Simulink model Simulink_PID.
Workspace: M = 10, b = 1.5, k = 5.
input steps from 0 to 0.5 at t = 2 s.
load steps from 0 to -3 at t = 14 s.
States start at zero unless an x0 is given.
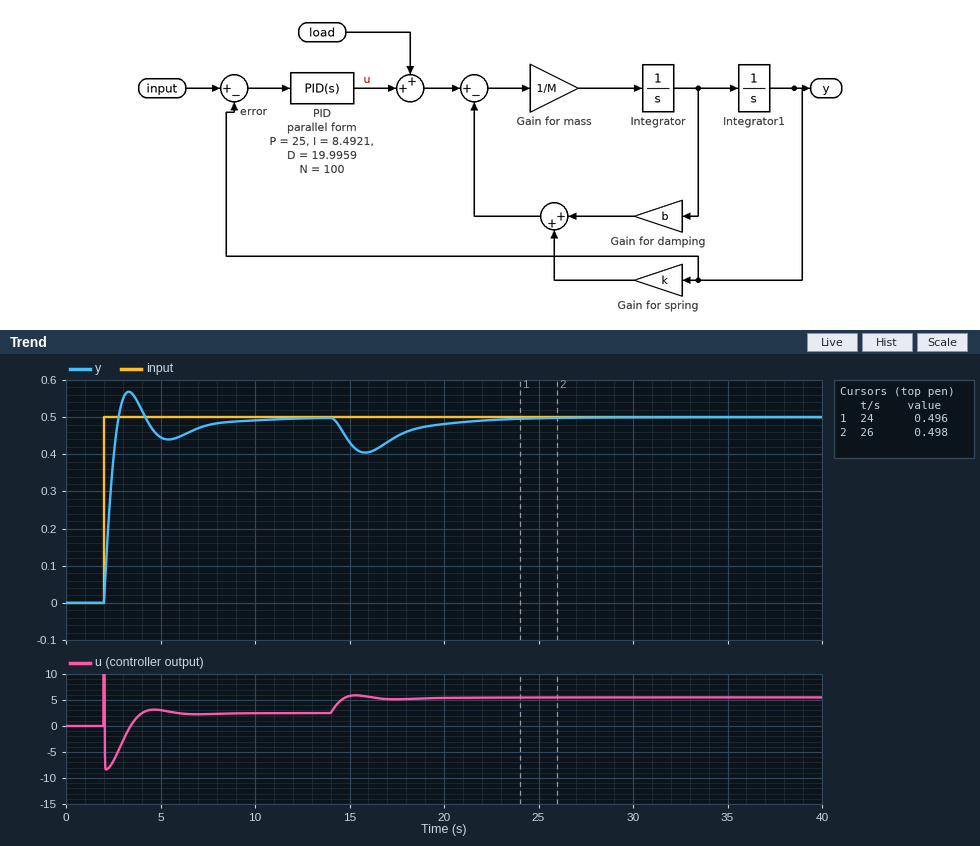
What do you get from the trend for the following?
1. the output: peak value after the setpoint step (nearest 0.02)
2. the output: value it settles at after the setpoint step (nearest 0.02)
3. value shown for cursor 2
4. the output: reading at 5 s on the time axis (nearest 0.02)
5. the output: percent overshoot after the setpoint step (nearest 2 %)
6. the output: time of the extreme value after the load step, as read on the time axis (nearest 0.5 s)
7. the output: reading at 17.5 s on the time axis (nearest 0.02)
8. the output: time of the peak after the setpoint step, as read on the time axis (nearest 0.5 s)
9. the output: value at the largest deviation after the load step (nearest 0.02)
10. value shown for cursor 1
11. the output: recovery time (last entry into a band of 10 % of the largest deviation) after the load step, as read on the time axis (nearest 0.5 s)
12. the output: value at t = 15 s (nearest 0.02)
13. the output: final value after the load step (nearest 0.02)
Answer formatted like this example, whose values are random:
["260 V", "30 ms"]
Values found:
["0.56", "0.50", "0.498", "0.44", "14 %", "16.0 s", "0.44", "3.5 s", "0.40", "0.496", "22.0 s", "0.44", "0.50"]
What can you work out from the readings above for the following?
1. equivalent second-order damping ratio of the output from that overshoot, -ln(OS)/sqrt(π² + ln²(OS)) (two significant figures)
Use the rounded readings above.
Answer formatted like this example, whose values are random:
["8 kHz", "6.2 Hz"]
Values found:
["0.53"]
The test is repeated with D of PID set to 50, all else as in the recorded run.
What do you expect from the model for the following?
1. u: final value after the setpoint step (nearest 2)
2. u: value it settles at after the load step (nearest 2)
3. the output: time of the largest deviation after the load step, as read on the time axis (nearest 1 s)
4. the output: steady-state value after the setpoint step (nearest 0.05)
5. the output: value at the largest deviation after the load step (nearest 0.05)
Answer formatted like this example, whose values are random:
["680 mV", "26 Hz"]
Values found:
["2", "6", "17 s", "0.50", "0.45"]
